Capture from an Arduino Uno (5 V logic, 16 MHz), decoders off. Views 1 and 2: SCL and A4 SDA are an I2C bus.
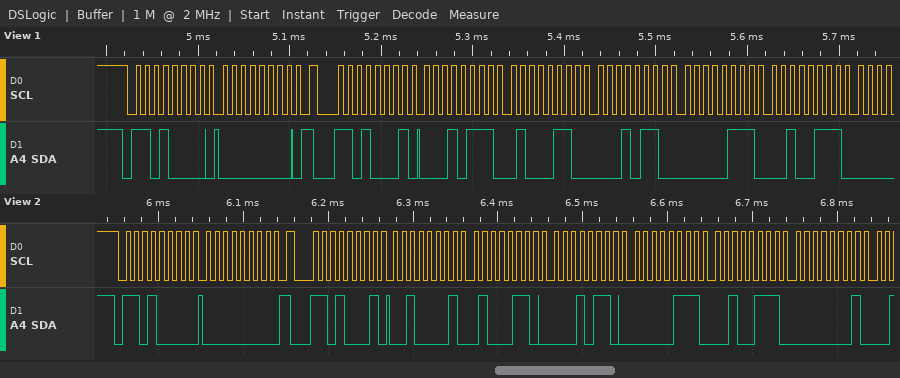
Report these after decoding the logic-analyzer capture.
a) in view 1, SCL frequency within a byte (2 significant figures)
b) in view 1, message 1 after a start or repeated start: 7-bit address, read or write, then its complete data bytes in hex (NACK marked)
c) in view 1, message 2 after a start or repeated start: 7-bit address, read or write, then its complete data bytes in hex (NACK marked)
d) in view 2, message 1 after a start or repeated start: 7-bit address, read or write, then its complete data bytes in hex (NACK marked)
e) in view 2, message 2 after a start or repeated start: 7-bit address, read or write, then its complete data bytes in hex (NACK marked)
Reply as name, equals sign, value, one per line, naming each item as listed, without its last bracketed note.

in view 1, SCL frequency within a byte = 100 kHz
in view 1, message 1 after a start or repeated start: 7-bit address, read or write, then its complete data bytes in hex = 0x68 write: 00
in view 1, message 2 after a start or repeated start: 7-bit address, read or write, then its complete data bytes in hex = 0x68 read: 17 46 16 07 27
in view 2, message 1 after a start or repeated start: 7-bit address, read or write, then its complete data bytes in hex = 0x68 write: 00
in view 2, message 2 after a start or repeated start: 7-bit address, read or write, then its complete data bytes in hex = 0x68 read: 21 46 16 07 27 01
